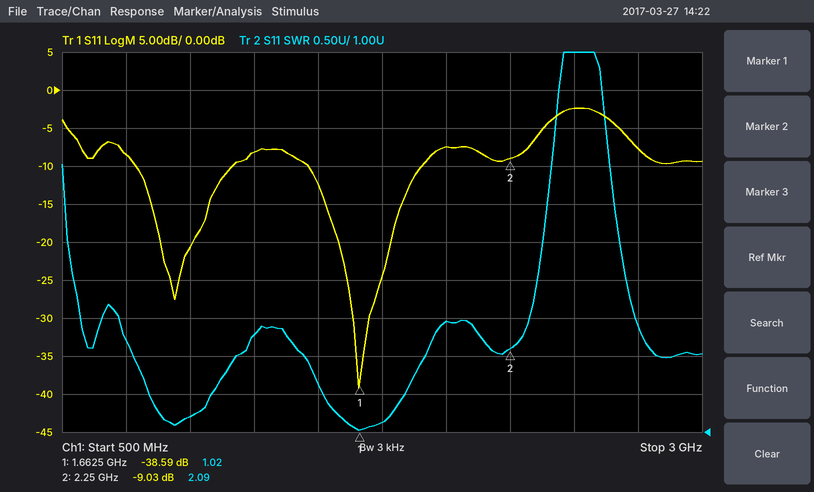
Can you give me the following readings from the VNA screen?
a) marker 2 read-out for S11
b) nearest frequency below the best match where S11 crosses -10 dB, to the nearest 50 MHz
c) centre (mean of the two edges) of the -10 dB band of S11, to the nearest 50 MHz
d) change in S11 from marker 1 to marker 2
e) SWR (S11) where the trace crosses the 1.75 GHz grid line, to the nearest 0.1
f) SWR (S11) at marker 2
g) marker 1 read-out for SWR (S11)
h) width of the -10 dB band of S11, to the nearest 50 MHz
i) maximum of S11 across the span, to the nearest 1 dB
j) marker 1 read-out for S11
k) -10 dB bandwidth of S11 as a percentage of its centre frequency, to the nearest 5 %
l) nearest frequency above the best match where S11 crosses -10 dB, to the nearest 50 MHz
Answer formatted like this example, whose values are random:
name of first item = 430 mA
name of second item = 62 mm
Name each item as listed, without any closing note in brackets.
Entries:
marker 2 read-out for S11 = -9.03 dB
nearest frequency below the best match where S11 crosses -10 dB, to the nearest 50 MHz = 1.45 GHz
centre (mean of the two edges) of the -10 dB band of S11, to the nearest 50 MHz = 1.70 GHz
change in S11 from marker 1 to marker 2 = 29.56 dB
SWR (S11) where the trace crosses the 1.75 GHz grid line, to the nearest 0.1 = 1.1
SWR (S11) at marker 2 = 2.09
marker 1 read-out for SWR = 1.02
width of the -10 dB band of S11, to the nearest 50 MHz = 450 MHz
maximum of S11 across the span, to the nearest 1 dB = -2 dB
marker 1 read-out for S11 = -38.59 dB
-10 dB bandwidth of S11 as a percentage of its centre frequency, to the nearest 5 % = 25 %
nearest frequency above the best match where S11 crosses -10 dB, to the nearest 50 MHz = 1.90 GHz
